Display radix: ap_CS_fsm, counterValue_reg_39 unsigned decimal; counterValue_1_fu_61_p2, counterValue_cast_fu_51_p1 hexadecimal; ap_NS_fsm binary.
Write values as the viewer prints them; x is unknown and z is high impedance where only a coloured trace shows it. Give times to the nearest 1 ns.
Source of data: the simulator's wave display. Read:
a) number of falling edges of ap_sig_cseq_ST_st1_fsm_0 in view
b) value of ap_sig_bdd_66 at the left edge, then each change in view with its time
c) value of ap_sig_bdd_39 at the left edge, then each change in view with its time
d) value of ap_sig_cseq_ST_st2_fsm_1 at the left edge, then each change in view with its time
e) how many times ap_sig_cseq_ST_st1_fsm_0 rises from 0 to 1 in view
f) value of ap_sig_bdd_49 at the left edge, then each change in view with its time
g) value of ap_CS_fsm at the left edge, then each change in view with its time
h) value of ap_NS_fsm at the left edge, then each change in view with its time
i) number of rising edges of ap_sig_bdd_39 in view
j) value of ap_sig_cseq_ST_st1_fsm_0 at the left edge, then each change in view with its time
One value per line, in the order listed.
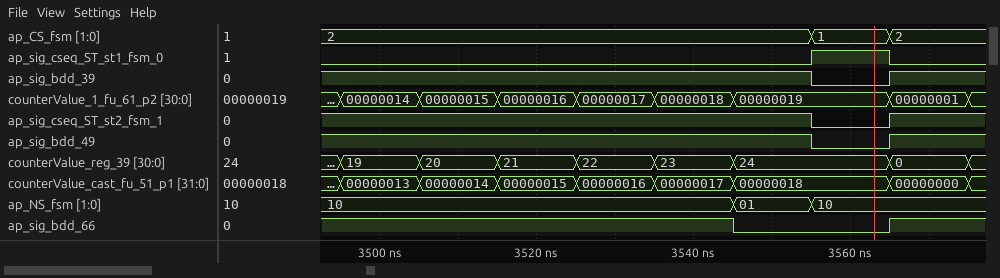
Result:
1
1, 0 at 3545 ns, 1 at 3565 ns
1, 0 at 3555 ns, 1 at 3565 ns
1, 0 at 3555 ns, 1 at 3565 ns
1
1, 0 at 3555 ns, 1 at 3565 ns
2, 1 at 3555 ns, 2 at 3565 ns
10, 01 at 3545 ns, 10 at 3555 ns
1
0, 1 at 3555 ns, 0 at 3565 ns
